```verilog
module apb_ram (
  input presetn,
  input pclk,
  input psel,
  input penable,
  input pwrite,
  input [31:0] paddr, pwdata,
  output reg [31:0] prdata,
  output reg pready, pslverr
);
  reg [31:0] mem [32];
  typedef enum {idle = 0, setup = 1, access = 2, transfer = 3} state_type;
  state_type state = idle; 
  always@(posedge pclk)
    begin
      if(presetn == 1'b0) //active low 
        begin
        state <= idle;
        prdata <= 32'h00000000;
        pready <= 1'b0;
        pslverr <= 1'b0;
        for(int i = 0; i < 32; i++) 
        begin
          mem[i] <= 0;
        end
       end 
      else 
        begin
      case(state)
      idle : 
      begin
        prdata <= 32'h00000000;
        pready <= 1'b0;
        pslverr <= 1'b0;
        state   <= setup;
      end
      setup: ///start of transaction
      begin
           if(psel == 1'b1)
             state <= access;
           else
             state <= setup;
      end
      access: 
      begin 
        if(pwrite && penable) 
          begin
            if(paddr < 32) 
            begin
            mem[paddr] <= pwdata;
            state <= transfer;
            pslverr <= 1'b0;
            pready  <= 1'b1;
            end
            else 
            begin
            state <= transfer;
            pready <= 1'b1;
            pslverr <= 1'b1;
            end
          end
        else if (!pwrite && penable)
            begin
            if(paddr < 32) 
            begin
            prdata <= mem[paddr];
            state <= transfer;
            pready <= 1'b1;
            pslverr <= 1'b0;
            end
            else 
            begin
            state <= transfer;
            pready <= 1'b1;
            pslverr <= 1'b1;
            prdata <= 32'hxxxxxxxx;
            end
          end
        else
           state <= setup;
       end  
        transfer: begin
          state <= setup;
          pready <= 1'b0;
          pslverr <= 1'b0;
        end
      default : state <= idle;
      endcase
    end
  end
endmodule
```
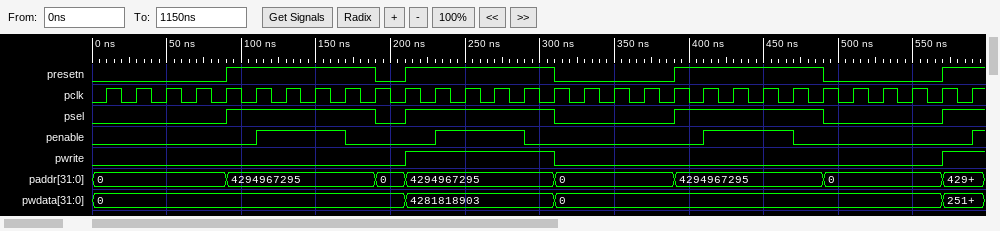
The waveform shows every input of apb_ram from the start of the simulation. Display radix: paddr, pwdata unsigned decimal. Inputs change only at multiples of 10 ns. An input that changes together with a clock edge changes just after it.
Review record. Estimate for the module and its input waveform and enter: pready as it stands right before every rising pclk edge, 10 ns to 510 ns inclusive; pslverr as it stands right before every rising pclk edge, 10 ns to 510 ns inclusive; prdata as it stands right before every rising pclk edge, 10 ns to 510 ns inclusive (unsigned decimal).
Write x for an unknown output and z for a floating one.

x 0 0 0 0 0 0 0 1 0 0 0 0 0 1 0 0 0 0 0 0 0 0 1 0 0
x 0 0 0 0 0 0 0 1 0 0 0 0 0 1 0 0 0 0 0 0 0 0 1 0 0
x, 0, 0, 0, 0, 0, 0, 0, x, x, x, 0, 0, 0, 0, 0, 0, 0, 0, 0, 0, 0, 0, x, x, x
